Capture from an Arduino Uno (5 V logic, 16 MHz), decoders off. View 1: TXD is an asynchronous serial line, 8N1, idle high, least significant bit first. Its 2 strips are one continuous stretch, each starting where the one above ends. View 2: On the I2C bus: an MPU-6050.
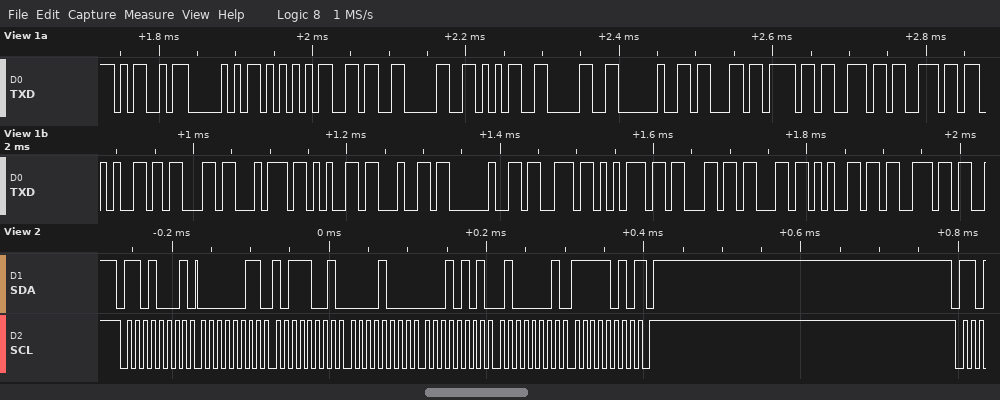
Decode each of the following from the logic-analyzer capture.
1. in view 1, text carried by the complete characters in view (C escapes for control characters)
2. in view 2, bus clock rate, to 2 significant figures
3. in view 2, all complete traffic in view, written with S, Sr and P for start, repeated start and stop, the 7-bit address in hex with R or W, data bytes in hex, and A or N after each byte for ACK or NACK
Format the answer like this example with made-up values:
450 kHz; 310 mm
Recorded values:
"MPU6050 connected succes"; 100 kHz; S 68R A 03 A B9 A 08 A 15 A 41 A FA N P
